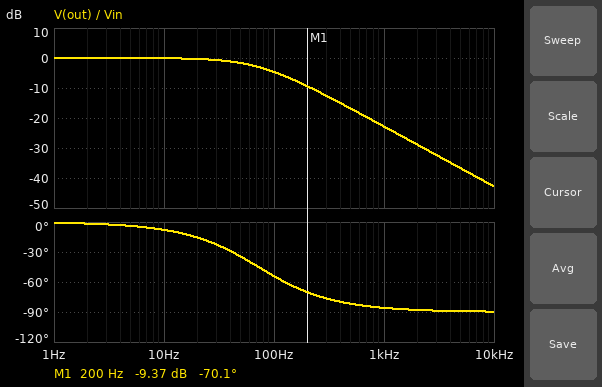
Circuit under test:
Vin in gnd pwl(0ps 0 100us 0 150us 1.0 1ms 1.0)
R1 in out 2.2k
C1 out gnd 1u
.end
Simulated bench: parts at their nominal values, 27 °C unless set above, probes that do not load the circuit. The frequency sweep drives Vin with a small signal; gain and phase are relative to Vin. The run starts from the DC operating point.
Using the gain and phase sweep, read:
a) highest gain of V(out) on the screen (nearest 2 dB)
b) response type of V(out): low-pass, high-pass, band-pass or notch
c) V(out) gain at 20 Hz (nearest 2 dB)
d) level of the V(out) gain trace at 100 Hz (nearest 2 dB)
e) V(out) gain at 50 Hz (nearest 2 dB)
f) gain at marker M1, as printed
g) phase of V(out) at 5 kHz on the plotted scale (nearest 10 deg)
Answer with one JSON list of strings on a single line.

["0 dB", "low-pass", "0 dB", "-4 dB", "-2 dB", "-9.37 dB", "-90 deg"]
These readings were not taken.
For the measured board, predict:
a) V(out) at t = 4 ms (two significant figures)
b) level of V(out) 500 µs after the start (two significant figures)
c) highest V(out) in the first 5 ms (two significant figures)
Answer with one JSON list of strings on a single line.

["830 mV", "160 mV", "890 mV"]
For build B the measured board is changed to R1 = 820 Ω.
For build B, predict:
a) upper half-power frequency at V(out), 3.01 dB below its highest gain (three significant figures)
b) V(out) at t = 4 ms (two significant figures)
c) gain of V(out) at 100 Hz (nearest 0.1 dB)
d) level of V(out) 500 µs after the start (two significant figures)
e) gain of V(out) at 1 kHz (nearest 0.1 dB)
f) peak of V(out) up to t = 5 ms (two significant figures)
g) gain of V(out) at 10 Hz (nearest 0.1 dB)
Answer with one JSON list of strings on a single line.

["194 Hz", "990 mV", "-1.0 dB", "370 mV", "-14.4 dB", "1.0 V", "0 dB"]
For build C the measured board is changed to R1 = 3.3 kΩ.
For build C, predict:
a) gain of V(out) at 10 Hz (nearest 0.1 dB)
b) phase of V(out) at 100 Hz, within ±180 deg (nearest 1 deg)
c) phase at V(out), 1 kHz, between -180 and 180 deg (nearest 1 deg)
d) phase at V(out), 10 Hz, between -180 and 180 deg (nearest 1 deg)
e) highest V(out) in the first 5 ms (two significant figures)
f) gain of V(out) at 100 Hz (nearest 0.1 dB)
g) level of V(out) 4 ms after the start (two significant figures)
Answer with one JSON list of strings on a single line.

["-0.2 dB", "-64 deg", "-87 deg", "-12 deg", "770 mV", "-7.2 dB", "690 mV"]
